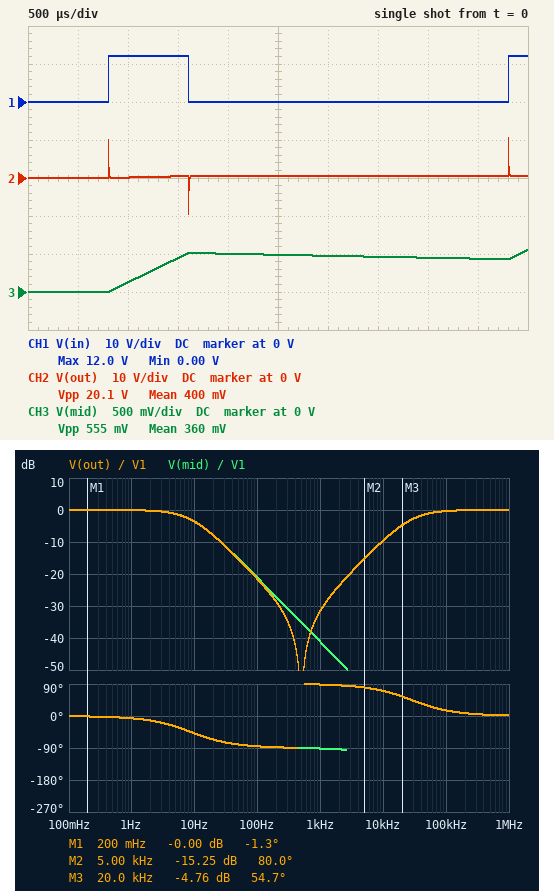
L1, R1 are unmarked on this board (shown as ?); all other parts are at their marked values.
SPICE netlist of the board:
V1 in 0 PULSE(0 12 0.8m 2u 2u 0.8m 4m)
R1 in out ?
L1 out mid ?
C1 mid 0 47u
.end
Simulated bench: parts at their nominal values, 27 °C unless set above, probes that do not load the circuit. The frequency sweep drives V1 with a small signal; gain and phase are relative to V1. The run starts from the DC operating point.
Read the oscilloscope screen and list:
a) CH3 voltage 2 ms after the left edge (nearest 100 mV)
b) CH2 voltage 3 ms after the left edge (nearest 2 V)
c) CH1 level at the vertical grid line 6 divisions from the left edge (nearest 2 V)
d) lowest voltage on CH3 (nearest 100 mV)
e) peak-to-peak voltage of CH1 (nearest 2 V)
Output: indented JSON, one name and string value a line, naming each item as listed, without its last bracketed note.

{
  "CH3 voltage 2 ms after the left edge": "500 mV",
  "CH2 voltage 3 ms after the left edge": "0 V",
  "CH1 level at the vertical grid line 6 divisions from the left edge": "0 V",
  "lowest voltage on CH3": "0 V",
  "peak-to-peak voltage of CH1": "12 V"
}
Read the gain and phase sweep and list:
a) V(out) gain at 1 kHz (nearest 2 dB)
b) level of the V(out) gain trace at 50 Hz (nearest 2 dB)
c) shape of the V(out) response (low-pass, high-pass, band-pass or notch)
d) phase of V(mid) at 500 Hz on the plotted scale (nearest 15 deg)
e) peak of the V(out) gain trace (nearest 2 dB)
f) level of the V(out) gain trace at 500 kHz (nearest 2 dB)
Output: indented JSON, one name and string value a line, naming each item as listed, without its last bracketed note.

{
  "V(out) gain at 1 kHz": "-32 dB",
  "level of the V(out) gain trace at 50 Hz": "-16 dB",
  "shape of the V(out) response": "notch",
  "phase of V(mid) at 500 Hz on the plotted scale": "-90 deg",
  "peak of the V(out) gain trace": "0 dB",
  "level of the V(out) gain trace at 500 kHz": "0 dB"
}
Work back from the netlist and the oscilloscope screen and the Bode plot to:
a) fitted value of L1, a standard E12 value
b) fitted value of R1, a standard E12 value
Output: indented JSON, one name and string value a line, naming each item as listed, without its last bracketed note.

{
  "fitted value of L1, a standard E12 value": "2.2 mH",
  "fitted value of R1, a standard E12 value": "390 Ω"
}
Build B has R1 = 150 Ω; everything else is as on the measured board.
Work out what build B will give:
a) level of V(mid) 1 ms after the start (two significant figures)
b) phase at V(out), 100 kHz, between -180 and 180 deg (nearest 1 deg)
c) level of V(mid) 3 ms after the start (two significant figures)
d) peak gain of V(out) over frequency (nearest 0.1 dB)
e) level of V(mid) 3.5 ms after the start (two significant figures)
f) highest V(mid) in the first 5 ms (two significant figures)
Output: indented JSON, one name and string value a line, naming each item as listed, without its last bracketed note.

{
  "level of V(mid) 1 ms after the start": "310 mV",
  "phase at V(out), 100 kHz, between -180 and 180 deg": "6 deg",
  "level of V(mid) 3 ms after the start": "1.1 V",
  "peak gain of V(out) over frequency": "0 dB",
  "level of V(mid) 3.5 ms after the start": "990 mV",
  "highest V(mid) in the first 5 ms": "1.3 V"
}
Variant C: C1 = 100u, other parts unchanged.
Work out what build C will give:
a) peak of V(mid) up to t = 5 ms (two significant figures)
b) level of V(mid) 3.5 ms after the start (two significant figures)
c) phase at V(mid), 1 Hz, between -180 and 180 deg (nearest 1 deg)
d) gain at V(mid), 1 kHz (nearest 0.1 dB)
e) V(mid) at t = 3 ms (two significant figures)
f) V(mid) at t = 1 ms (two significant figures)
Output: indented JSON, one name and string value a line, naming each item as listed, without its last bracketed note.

{
  "peak of V(mid) up to t = 5 ms": "280 mV",
  "level of V(mid) 3.5 ms after the start": "230 mV",
  "phase at V(mid), 1 Hz, between -180 and 180 deg": "-14 deg",
  "gain at V(mid), 1 kHz": "-47.8 dB",
  "V(mid) at t = 3 ms": "240 mV",
  "V(mid) at t = 1 ms": "59 mV"
}
